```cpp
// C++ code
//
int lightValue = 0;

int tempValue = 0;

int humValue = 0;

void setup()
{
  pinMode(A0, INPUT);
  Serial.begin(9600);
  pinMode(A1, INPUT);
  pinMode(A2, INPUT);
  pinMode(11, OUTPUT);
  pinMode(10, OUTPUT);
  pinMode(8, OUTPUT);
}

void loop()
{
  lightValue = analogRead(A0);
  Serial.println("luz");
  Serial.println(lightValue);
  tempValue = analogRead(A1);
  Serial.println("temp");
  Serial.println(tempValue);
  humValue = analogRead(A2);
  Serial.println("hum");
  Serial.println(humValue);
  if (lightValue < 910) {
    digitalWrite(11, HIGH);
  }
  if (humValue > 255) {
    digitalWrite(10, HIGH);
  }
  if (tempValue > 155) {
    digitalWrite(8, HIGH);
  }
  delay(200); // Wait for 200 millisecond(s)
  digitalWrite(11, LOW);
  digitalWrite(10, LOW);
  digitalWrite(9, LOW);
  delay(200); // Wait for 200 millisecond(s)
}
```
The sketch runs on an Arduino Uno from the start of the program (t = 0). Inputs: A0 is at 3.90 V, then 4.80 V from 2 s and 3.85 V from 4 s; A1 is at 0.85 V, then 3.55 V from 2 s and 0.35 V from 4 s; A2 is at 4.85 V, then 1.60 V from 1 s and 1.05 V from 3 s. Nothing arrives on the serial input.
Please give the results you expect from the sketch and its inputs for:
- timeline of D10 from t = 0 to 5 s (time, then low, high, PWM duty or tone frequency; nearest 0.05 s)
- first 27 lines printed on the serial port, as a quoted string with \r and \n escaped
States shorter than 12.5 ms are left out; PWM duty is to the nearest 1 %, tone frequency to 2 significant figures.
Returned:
0 s high; 0.2 s low; 0.4 s high; 0.6 s low; 0.8 s high; 1 s low; 1.2 s high; 1.4 s low; 1.6 s high; 1.8 s low; 2 s high; 2.2 s low; 2.4 s high; 2.6 s low; 2.8 s high; 3 s low
"luz\r\n798\r\ntemp\r\n174\r\nhum\r\n993\r\nluz\r\n798\r\ntemp\r\n174\r\nhum\r\n993\r\nluz\r\n798\r\ntemp\r\n174\r\nhum\r\n993\r\nluz\r\n798\r\ntemp\r\n174\r\nhum\r\n327\r\nluz\r\n798\r\ntemp\r\n"
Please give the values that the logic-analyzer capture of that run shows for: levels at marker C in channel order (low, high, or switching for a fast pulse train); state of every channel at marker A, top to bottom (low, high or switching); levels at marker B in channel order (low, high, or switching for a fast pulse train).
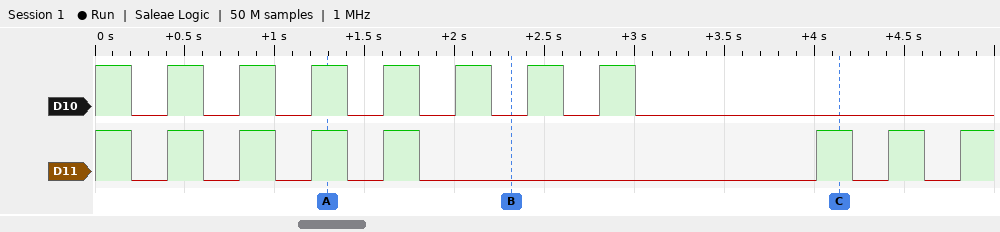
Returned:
D10 low, D11 high
D10 high, D11 high
D10 low, D11 low
